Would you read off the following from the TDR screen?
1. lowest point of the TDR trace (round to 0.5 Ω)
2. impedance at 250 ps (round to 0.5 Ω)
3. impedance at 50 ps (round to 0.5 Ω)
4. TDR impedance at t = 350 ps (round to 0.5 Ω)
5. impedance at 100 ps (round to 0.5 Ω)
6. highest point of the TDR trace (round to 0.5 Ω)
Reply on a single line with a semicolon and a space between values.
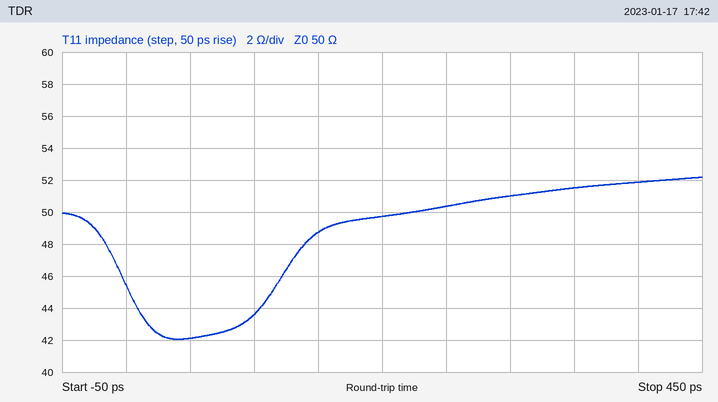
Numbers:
42.0 Ω; 50.5 Ω; 42.0 Ω; 51.5 Ω; 43.5 Ω; 52.0 Ω
